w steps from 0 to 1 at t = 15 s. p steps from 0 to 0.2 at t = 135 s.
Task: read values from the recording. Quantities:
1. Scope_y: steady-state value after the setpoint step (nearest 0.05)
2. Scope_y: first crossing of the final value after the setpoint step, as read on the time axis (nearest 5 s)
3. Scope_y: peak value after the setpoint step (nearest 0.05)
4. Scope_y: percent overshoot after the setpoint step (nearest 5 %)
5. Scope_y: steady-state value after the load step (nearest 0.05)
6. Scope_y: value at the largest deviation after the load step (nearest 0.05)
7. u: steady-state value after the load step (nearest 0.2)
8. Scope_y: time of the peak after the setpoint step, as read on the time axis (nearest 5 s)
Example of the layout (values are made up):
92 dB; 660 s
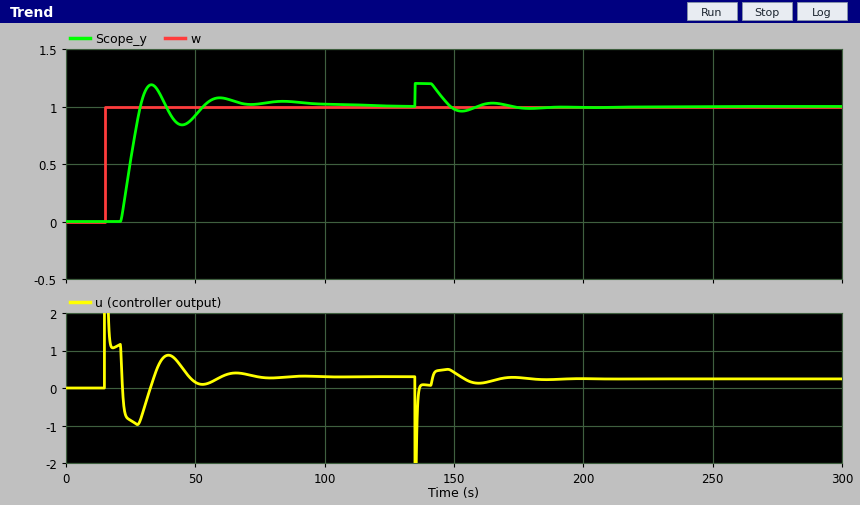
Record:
1.00; 30 s; 1.20; 20 %; 1.00; 1.20; 0.2; 35 s
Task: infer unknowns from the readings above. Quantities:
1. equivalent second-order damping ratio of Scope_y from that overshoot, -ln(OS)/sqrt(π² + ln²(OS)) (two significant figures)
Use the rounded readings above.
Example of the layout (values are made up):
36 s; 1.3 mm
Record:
0.46
